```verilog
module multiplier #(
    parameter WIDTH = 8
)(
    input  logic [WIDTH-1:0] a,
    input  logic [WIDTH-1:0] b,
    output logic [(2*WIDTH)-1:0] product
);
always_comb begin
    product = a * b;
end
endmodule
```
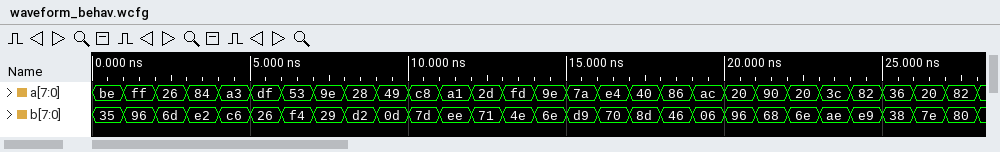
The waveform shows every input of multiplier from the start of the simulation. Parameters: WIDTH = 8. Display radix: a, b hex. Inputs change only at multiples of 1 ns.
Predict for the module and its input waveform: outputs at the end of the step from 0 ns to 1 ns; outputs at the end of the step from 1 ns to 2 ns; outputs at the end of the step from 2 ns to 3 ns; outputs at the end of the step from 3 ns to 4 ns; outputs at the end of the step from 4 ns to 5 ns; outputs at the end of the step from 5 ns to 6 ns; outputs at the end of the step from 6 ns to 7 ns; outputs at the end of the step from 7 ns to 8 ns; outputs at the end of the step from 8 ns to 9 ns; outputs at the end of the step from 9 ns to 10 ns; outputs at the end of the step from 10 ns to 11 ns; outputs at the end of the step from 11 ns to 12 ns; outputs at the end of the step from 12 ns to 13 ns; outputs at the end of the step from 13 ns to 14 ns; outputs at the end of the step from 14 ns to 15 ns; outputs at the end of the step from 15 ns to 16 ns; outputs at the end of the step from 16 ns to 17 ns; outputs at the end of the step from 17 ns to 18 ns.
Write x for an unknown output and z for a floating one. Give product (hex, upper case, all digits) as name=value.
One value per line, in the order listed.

product=2756
product=956A
product=102E
product=7488
product=7E12
product=211A
product=4F1C
product=194E
product=20D0
product=03B5
product=61A8
product=95AE
product=13DD
product=4D16
product=43E4
product=676A
product=63C0
product=2340
